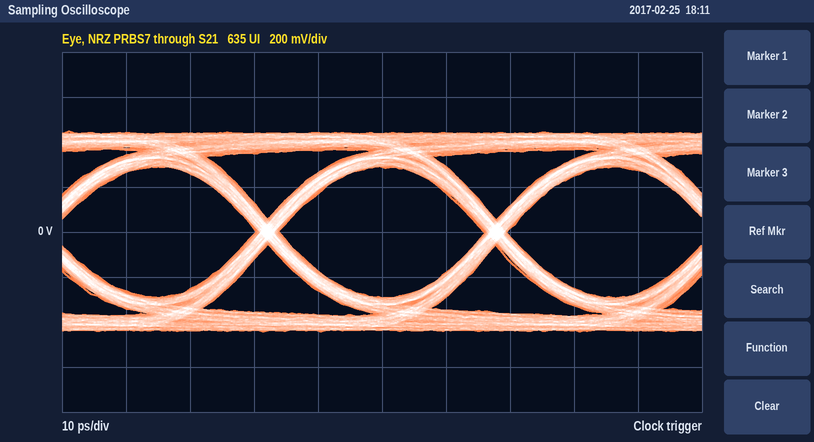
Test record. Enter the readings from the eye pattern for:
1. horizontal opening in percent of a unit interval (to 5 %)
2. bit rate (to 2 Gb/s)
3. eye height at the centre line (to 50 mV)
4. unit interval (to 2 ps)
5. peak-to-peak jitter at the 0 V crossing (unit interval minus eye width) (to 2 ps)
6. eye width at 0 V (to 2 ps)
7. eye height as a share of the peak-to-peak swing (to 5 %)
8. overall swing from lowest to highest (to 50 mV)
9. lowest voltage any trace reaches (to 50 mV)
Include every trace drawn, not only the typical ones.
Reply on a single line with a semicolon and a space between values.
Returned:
90 %; 28 Gb/s; 600 mV; 36 ps; 4 ps; 32 ps; 65 %; 900 mV; -450 mV
